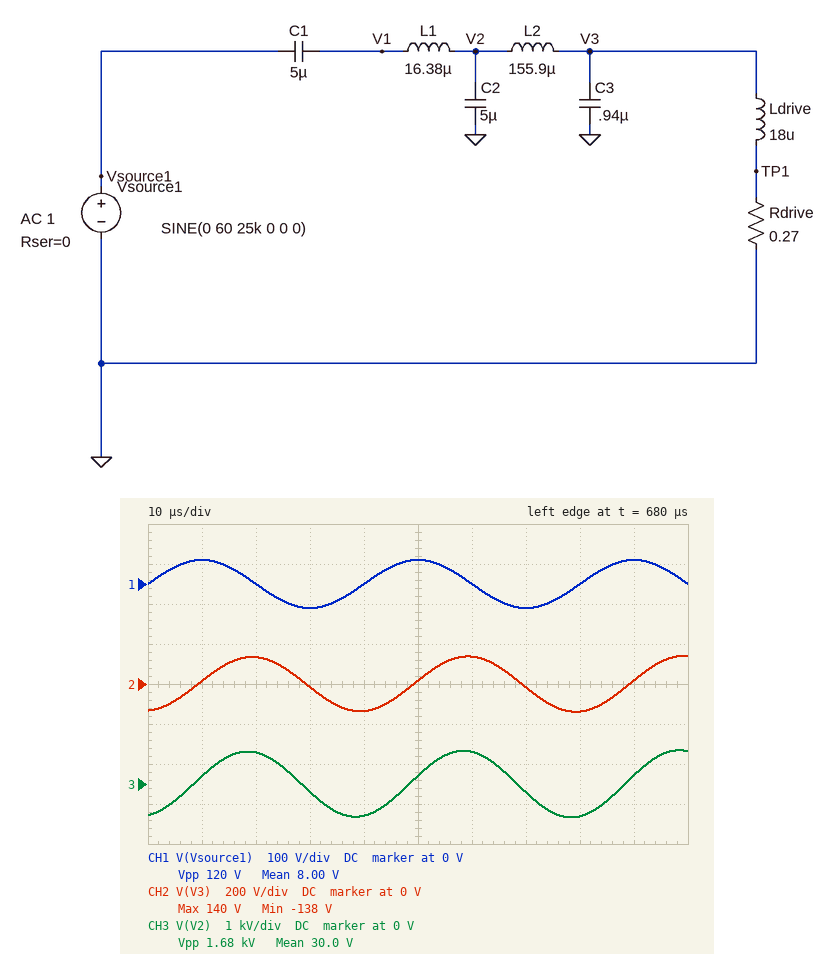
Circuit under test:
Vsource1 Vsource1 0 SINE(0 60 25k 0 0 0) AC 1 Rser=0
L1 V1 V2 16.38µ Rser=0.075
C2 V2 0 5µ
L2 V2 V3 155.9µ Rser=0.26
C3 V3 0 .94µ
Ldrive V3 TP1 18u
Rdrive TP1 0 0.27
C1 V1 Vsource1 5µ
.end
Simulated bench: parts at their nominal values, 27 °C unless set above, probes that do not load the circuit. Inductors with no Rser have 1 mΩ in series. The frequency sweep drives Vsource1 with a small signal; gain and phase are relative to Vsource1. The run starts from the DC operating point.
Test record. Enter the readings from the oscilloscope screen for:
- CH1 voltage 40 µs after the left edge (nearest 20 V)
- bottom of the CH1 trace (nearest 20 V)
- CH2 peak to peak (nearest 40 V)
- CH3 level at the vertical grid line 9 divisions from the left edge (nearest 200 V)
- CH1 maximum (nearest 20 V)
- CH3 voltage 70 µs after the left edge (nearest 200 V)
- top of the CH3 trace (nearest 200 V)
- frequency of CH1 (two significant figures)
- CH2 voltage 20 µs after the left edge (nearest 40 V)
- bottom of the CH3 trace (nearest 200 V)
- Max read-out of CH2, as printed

0 V
-60 V
280 V
200 V
60 V
-200 V
800 V
25 kHz
120 V
-800 V
140 V
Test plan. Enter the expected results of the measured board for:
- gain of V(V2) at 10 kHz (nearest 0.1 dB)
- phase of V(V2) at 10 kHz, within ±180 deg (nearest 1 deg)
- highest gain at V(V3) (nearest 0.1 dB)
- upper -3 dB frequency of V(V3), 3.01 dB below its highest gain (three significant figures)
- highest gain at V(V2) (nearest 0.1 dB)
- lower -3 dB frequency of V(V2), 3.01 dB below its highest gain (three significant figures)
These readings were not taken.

-3.4 dB
0 deg
9.1 dB
25.5 kHz
24.7 dB
24.8 kHz
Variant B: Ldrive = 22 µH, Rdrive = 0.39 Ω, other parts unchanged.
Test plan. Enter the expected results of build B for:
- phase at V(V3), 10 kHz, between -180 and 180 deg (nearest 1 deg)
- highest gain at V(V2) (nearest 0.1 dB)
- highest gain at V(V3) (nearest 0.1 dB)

-14 deg
24.5 dB
11.6 dB
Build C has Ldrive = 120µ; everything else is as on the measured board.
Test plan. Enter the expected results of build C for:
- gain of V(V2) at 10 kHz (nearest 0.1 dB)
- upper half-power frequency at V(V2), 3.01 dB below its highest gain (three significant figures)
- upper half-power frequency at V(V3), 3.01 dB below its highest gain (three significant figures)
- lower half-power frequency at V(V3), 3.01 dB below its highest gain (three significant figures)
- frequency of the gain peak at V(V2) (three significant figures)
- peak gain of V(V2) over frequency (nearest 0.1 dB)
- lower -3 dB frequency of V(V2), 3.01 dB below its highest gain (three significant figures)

-4.0 dB
25.8 kHz
20.0 kHz
19.6 kHz
25.4 kHz
24.9 dB
25.1 kHz
